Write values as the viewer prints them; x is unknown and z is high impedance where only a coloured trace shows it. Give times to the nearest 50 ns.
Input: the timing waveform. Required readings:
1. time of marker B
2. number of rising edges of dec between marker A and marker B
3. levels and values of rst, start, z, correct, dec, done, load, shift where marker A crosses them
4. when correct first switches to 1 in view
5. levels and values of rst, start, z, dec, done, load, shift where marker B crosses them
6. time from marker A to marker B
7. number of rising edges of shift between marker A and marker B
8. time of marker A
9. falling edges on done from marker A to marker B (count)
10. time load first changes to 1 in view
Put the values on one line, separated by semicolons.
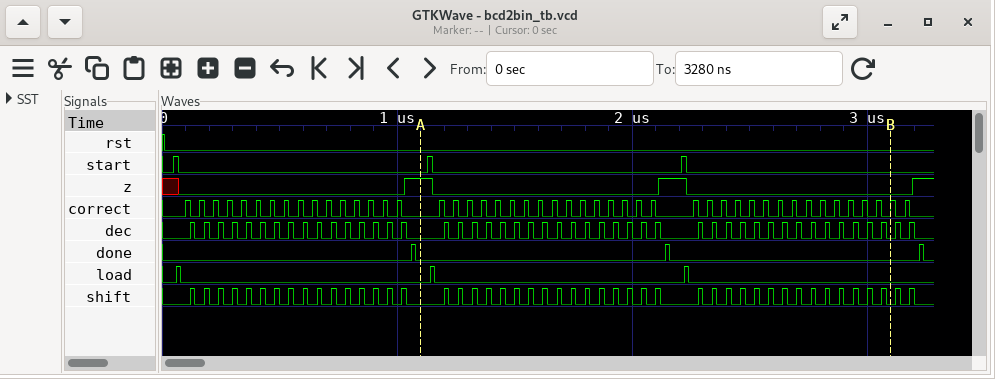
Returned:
3100 ns; 30; rst=0, start=0, z=1, correct=0, dec=0, done=0, load=0, shift=0; 100 ns; rst=0, start=0, z=0, dec=0, done=0, load=0, shift=0; 2000 ns; 30; 1100 ns; 1; 50 ns
